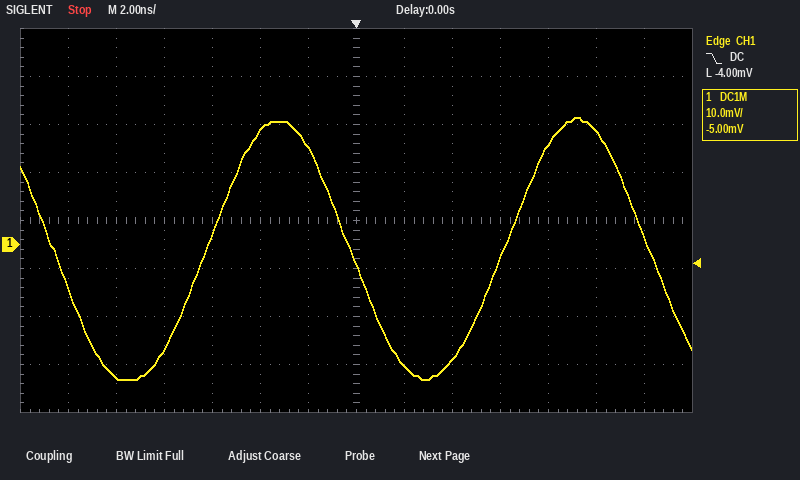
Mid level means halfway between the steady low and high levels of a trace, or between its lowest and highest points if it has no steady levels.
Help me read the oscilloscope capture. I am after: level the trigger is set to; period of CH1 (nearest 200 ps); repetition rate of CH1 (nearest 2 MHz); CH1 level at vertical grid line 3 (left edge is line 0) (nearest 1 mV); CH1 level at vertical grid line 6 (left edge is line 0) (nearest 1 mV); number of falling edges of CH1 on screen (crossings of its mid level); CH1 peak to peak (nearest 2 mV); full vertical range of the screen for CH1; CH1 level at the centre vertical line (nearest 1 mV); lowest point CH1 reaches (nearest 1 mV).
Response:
-4.00 mV
12.4 ns
80 MHz
-22 mV
20 mV
3
54 mV
80 mV
-4 mV
-28 mV
